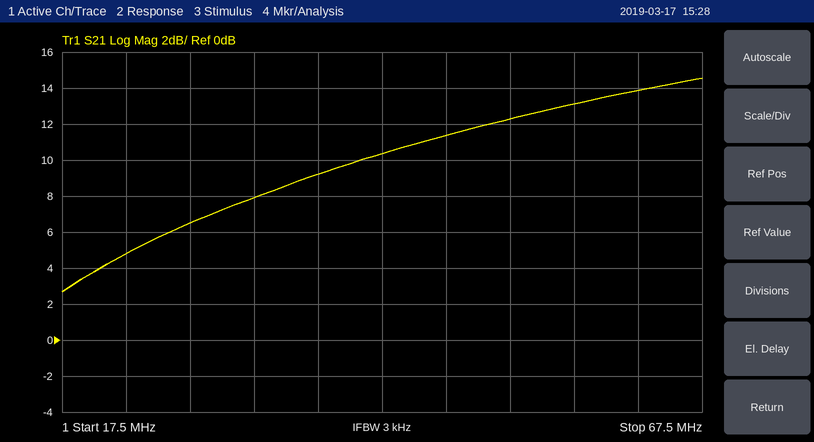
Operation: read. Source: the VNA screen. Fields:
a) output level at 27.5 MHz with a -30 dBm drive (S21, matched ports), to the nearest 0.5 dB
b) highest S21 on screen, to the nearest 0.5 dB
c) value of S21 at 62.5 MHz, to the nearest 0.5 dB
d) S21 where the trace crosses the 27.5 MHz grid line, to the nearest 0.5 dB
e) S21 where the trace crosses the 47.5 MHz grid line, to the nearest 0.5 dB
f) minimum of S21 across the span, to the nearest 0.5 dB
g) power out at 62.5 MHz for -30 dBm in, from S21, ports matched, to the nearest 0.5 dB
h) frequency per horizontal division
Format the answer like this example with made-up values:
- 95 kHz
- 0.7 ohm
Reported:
- -23.5 dBm
- 14.5 dB
- 14.0 dB
- 6.5 dB
- 11.5 dB
- 2.5 dB
- -16.0 dBm
- 5 MHz
